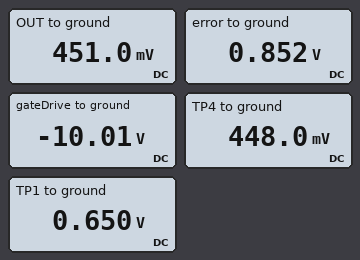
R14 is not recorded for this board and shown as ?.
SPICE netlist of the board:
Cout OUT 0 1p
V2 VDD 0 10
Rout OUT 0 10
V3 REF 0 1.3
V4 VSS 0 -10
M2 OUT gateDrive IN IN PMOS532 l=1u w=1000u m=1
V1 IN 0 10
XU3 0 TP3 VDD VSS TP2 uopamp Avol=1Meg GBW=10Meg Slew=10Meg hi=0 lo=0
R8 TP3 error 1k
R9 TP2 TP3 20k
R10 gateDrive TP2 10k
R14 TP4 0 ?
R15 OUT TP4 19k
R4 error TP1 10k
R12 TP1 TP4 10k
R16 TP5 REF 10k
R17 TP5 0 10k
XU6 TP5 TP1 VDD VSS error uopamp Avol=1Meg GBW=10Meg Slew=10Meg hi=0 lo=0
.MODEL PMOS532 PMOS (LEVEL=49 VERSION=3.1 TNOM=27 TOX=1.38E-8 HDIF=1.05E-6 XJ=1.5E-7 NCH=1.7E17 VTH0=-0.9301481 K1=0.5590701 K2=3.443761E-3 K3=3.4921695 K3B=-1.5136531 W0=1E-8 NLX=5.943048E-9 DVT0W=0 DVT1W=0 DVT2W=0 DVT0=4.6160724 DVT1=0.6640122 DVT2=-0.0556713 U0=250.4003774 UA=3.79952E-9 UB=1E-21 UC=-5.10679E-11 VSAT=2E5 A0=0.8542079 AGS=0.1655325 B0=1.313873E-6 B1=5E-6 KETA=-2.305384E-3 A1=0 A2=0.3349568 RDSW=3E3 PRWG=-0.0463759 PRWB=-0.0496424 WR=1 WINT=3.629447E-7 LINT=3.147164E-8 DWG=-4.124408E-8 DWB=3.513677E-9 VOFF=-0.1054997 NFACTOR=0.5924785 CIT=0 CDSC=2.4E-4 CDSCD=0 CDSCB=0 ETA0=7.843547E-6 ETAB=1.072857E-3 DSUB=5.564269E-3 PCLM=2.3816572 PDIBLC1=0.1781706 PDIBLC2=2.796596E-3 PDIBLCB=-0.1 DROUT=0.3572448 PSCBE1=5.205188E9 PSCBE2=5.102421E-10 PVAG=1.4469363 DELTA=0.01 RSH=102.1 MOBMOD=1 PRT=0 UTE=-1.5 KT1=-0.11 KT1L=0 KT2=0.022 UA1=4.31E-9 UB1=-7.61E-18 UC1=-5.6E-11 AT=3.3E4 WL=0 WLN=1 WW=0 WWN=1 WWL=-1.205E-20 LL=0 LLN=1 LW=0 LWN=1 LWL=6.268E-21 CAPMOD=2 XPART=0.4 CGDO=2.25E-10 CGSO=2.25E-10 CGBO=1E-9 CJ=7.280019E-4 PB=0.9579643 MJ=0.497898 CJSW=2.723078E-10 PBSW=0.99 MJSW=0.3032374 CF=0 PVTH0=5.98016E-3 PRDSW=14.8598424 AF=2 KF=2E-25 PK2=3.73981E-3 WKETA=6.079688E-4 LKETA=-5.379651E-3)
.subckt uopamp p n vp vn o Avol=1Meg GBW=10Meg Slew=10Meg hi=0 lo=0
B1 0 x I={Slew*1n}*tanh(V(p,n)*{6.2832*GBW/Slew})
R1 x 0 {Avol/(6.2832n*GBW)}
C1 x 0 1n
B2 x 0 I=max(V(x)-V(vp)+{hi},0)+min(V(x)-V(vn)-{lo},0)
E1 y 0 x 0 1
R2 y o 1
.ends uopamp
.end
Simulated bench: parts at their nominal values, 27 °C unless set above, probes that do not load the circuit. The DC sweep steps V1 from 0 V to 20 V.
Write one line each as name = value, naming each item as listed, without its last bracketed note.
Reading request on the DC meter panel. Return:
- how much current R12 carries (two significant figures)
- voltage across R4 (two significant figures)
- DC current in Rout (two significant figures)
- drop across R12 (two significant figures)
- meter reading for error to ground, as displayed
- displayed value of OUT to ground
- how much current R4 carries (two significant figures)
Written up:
how much current R12 carries = 20 µA
voltage across R4 = 200 mV
DC current in Rout = 45 mA
drop across R12 = 200 mV
meter reading for error to ground, as displayed = 0.852 V
displayed value of OUT to ground = 451.0 mV
how much current R4 carries = 20 µA
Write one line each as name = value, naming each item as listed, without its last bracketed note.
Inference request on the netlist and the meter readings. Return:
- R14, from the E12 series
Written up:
R14, from the E12 series = 22 kΩ
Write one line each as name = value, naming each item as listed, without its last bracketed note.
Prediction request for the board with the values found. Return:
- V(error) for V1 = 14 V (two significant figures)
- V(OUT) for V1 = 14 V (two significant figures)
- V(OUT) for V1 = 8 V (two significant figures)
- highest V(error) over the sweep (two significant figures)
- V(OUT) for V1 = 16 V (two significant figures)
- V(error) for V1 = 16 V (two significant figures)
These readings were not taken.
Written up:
V(error) for V1 = 14 V = 800 mV
V(OUT) for V1 = 14 V = 630 mV
V(OUT) for V1 = 8 V = 360 mV
highest V(error) over the sweep = 970 mV
V(OUT) for V1 = 16 V = 720 mV
V(error) for V1 = 16 V = 780 mV
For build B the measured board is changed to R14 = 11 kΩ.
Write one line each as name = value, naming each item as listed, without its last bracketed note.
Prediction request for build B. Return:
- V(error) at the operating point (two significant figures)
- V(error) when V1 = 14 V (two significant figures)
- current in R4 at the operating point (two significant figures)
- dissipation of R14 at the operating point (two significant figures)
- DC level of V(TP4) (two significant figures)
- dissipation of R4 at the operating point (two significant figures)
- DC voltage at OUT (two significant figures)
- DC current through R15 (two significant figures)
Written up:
V(error) at the operating point = 940 mV
V(error) when V1 = 14 V = 900 mV
current in R4 at the operating point = 29 µA
dissipation of R14 at the operating point = 12 µW
DC level of V(TP4) = 360 mV
dissipation of R4 at the operating point = 8.2 µW
DC voltage at OUT = 450 mV
DC current through R15 = 4.6 µA
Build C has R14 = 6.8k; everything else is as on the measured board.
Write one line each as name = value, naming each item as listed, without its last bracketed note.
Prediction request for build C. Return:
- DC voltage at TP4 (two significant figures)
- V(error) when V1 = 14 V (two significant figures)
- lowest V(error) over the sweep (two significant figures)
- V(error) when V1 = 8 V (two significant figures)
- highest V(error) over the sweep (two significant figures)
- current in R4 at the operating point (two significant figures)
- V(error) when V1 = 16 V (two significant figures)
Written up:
DC voltage at TP4 = 300 mV
V(error) when V1 = 14 V = 970 mV
lowest V(error) over the sweep = 920 mV
V(error) when V1 = 8 V = 1.0 V
highest V(error) over the sweep = 1.1 V
current in R4 at the operating point = 35 µA
V(error) when V1 = 16 V = 960 mV
